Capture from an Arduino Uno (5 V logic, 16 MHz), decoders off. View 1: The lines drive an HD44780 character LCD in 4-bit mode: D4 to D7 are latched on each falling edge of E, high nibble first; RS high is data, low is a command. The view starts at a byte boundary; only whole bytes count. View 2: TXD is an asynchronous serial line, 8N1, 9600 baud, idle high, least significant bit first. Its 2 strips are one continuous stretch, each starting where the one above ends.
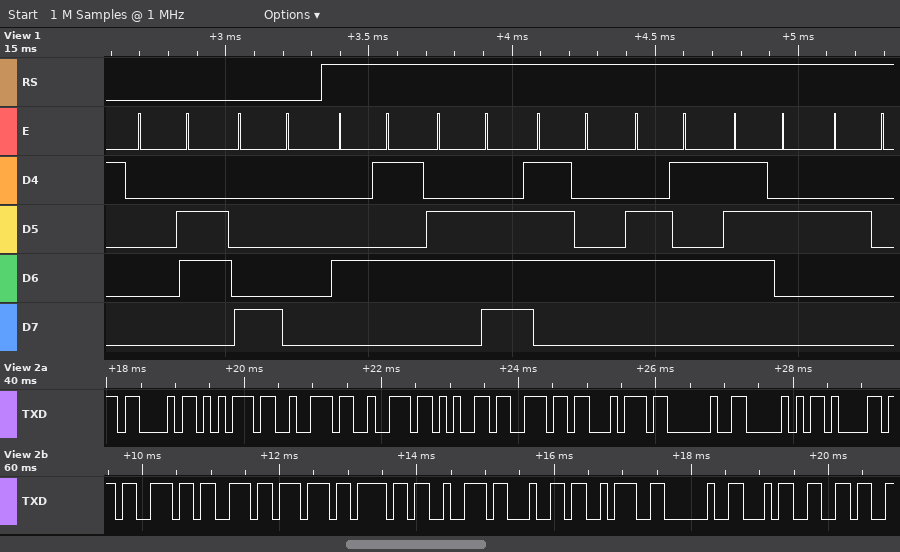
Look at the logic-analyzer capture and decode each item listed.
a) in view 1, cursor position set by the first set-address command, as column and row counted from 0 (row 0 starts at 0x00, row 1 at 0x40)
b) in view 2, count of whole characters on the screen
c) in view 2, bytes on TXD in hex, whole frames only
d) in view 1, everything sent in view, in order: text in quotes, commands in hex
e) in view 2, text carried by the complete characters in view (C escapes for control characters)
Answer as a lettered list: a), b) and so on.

a) column 0, row 0
b) 20
c) 43 75 72 72 65 6E 74 20 50 61 73 73 77 6F 72 64 3A 20 34 36
d) 0x06 0x80 "Enter "
e) "Current Password: 46"
